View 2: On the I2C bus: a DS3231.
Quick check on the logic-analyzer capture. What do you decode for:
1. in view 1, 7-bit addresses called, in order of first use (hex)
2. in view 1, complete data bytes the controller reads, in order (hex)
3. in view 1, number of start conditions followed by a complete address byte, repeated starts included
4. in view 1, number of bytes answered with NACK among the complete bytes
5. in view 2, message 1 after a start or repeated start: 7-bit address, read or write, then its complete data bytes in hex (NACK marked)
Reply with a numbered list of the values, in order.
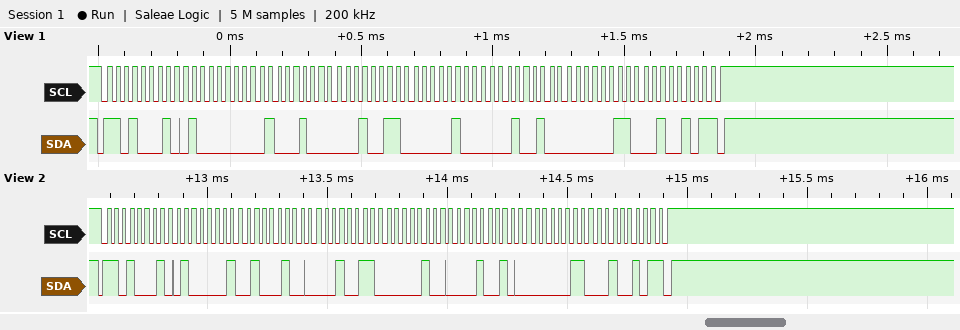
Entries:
1. 0x68
2. 40 44 13 04 12 03 25
3. 1
4. 1
5. 0x68 read: 41 44 13 04 12 03 25 NACK
